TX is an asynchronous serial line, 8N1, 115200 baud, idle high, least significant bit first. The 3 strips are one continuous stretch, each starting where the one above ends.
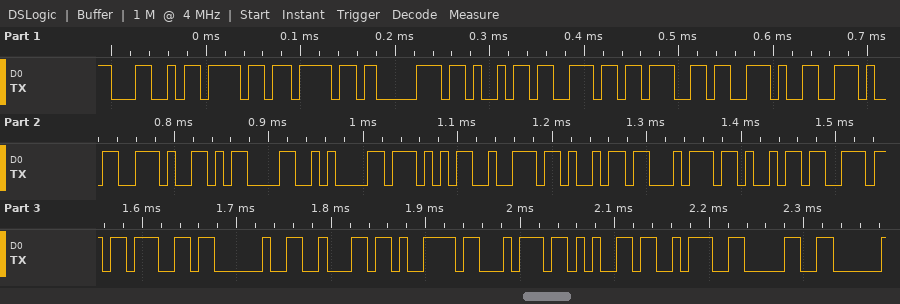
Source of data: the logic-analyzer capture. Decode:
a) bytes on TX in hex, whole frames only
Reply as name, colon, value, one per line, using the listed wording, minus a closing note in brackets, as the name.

bytes on TX in hex, whole frames only: 0x4C 0x6F 0x6F 0x70 0x69 0x6E 0x67 0x2E 0x2E 0x2E 0x0D 0x0A 0x57 0x72 0x69 0x74 0x69 0x6E 0x67 0x20 0x62 0x79 0x74 0x65 0x3A 0x30
